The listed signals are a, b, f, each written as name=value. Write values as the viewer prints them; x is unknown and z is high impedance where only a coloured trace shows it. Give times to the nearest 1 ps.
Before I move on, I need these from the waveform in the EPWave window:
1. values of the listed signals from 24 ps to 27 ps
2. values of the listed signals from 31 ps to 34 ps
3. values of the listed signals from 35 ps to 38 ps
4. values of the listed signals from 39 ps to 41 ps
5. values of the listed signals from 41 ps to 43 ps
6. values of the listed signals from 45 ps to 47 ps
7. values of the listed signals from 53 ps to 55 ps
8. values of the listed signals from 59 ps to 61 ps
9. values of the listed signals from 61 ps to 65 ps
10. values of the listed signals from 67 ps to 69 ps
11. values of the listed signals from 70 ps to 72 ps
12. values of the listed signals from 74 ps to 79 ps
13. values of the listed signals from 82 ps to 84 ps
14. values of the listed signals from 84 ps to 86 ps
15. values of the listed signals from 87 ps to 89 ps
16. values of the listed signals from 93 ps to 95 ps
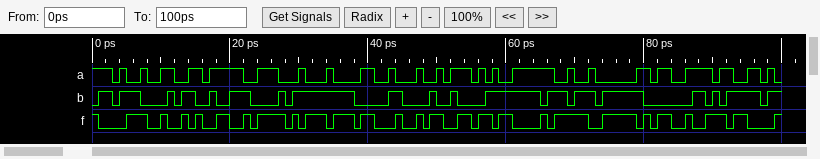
a=1, b=0, f=1
a=0, b=1, f=1
a=0, b=1, f=1
a=1, b=0, f=1
a=0, b=0, f=0
a=0, b=0, f=0
a=1, b=0, f=1
a=0, b=1, f=1
a=1, b=1, f=0
a=0, b=1, f=1
a=0, b=1, f=1
a=0, b=1, f=1
a=1, b=0, f=1
a=0, b=0, f=0
a=1, b=1, f=0
a=0, b=1, f=1
